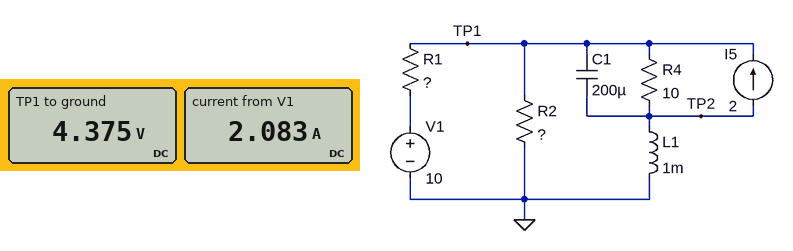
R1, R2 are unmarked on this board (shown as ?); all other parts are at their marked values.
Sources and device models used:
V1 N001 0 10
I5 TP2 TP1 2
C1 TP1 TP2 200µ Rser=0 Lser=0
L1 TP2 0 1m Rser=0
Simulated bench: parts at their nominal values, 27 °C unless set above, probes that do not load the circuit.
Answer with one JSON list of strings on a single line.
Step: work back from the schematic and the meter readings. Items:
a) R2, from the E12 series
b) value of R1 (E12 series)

["1.2 Ω", "2.7 Ω"]
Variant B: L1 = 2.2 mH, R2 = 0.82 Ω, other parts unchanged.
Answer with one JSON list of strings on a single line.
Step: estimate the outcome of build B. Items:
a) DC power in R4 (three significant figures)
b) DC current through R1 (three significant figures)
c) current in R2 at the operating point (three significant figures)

["1.14 W", "2.45 A", "4.12 A"]
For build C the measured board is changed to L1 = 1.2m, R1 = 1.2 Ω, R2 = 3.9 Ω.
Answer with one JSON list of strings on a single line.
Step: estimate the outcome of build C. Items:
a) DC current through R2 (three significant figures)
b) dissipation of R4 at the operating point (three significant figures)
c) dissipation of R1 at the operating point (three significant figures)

["2.23 A", "7.54 W", "1.44 W"]
